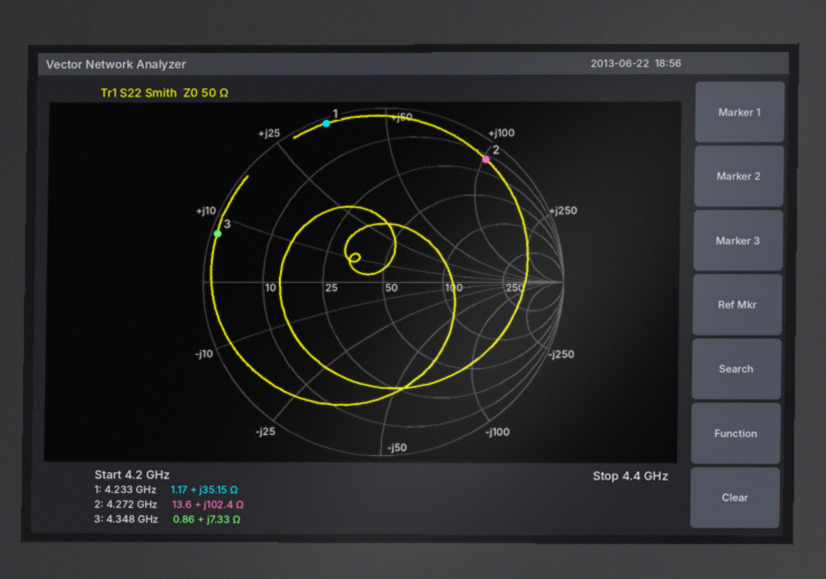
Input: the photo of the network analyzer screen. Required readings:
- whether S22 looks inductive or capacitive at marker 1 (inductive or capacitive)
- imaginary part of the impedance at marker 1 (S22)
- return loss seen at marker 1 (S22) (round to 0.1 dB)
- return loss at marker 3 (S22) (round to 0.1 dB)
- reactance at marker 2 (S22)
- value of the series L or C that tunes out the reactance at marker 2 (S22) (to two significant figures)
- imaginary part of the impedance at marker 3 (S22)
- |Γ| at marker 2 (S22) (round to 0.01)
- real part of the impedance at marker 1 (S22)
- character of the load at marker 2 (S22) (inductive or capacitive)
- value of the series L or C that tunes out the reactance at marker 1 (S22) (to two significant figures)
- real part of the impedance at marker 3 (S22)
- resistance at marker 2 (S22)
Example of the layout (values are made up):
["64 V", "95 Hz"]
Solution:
["inductive", "+35.15 Ω", "0.3 dB", "0.3 dB", "+102.4 Ω", "360 fF", "+7.33 Ω", "0.90", "1.17 Ω", "inductive", "1.1 pF", "0.86 Ω", "13.6 Ω"]
